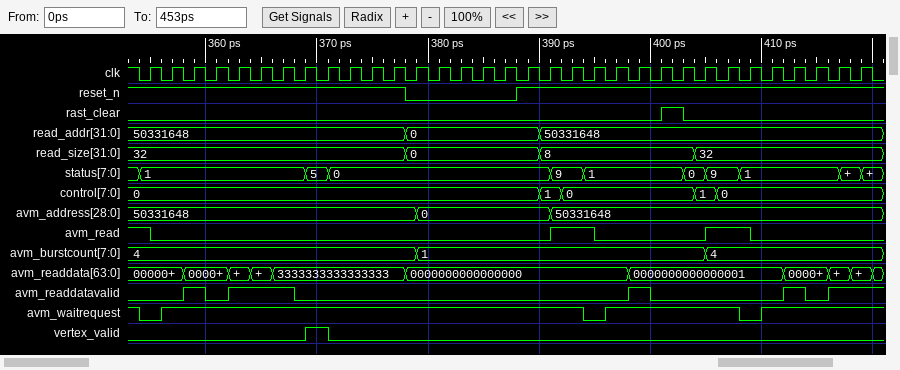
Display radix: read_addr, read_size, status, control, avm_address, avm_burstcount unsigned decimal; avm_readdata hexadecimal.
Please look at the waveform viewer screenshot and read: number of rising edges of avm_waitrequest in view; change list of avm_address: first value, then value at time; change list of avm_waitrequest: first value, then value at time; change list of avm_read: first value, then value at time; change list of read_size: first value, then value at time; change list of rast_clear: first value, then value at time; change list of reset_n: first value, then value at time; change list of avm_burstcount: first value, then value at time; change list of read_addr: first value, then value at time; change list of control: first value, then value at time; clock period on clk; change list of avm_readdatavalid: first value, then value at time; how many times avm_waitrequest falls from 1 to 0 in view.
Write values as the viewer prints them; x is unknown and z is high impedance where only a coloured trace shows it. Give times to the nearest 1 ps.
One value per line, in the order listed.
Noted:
3
50331648, 0 at 379 ps, 50331648 at 391 ps
1, 0 at 354 ps, 1 at 356 ps, 0 at 394 ps, 1 at 396 ps, 0 at 408 ps, 1 at 410 ps
1, 0 at 355 ps, 1 at 391 ps, 0 at 395 ps, 1 at 405 ps, 0 at 409 ps
32, 0 at 378 ps, 8 at 390 ps, 32 at 404 ps
0, 1 at 401 ps, 0 at 403 ps
1, 0 at 378 ps, 1 at 388 ps
4, 1 at 379 ps, 4 at 405 ps
50331648, 0 at 378 ps, 50331648 at 390 ps
0, 1 at 390 ps, 0 at 392 ps, 1 at 404 ps, 0 at 406 ps
2 ps
0, 1 at 358 ps, 0 at 360 ps, 1 at 362 ps, 0 at 368 ps, 1 at 398 ps, 0 at 400 ps, 1 at 412 ps, 0 at 414 ps, 1 at 416 ps
3
